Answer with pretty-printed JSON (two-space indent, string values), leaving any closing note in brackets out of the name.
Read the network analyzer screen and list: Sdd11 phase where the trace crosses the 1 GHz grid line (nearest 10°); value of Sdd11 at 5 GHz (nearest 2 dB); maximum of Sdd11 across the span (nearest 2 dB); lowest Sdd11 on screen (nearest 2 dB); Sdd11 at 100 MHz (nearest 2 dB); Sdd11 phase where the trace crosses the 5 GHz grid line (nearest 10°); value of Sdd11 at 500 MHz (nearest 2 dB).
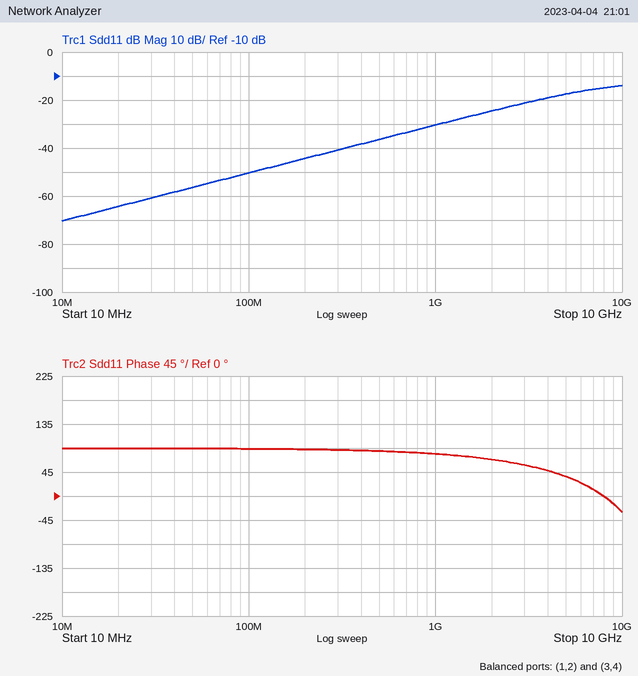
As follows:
{
  "Sdd11 phase where the trace crosses the 1 GHz grid line": "80°",
  "value of Sdd11 at 5 GHz": "-18 dB",
  "maximum of Sdd11 across the span": "-14 dB",
  "lowest Sdd11 on screen": "-70 dB",
  "Sdd11 at 100 MHz": "-50 dB",
  "Sdd11 phase where the trace crosses the 5 GHz grid line": "40°",
  "value of Sdd11 at 500 MHz": "-36 dB"
}
